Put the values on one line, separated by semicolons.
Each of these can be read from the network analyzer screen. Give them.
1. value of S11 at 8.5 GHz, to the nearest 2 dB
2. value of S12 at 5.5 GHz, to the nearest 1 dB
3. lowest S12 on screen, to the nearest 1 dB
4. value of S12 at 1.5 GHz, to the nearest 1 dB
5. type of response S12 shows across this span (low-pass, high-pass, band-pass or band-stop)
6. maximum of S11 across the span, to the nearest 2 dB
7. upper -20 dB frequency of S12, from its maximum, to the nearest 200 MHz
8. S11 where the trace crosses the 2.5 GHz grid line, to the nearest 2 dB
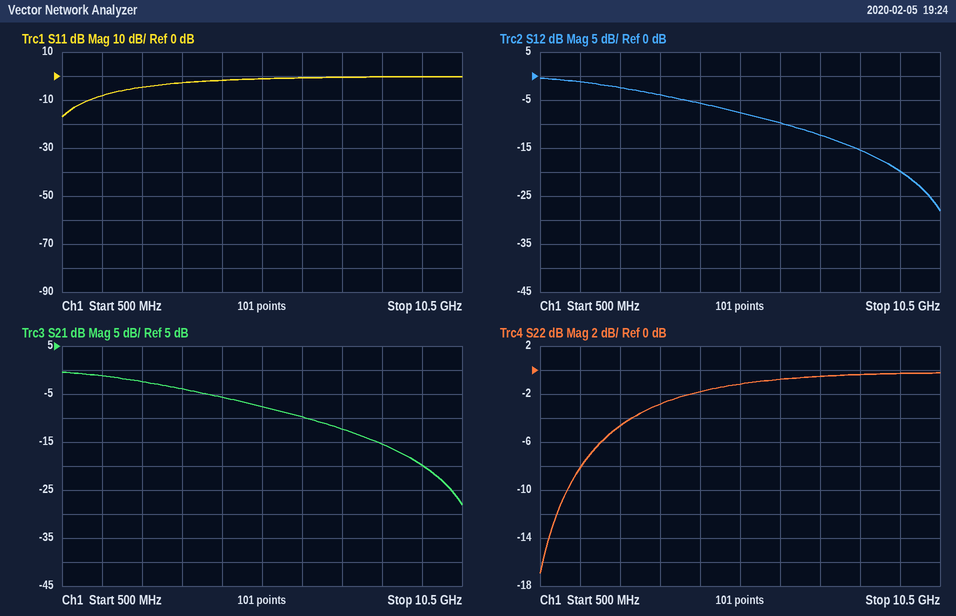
0 dB; -8 dB; -28 dB; -1 dB; low-pass; 0 dB; 9.6 GHz; -4 dB
